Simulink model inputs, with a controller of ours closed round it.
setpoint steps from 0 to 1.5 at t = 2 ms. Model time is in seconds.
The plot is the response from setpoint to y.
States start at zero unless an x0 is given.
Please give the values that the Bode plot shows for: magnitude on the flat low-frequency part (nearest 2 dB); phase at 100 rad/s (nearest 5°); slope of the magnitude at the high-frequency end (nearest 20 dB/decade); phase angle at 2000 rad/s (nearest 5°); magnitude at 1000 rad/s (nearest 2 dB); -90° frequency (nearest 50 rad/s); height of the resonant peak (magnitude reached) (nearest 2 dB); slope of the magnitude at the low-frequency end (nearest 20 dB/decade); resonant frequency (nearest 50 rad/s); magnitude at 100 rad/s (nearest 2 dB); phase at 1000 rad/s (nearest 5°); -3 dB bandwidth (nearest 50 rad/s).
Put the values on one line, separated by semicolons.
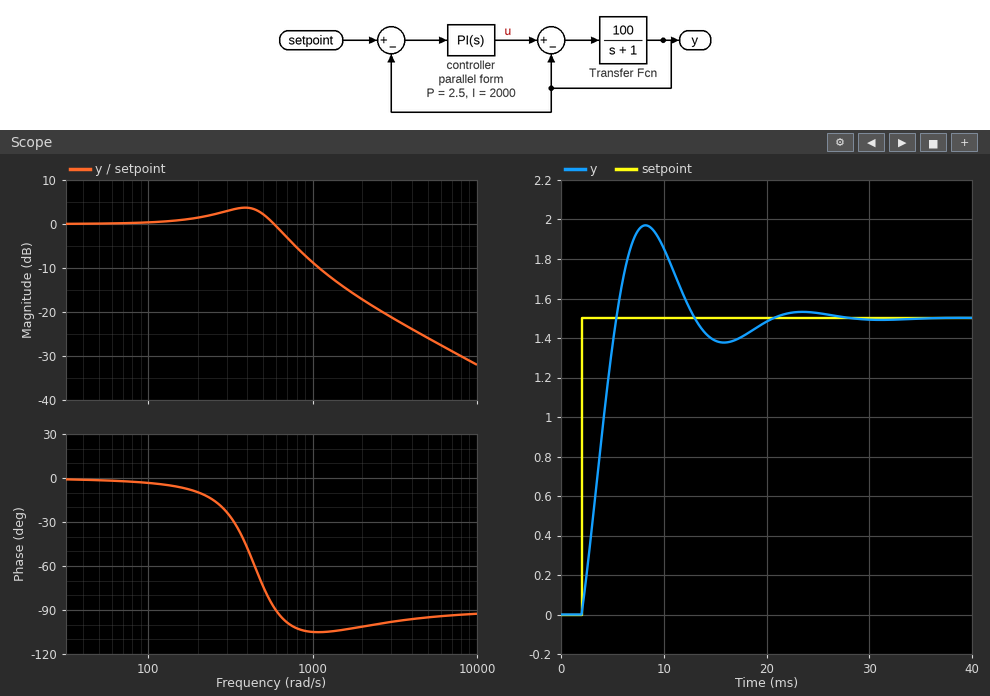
0 dB; -5°; -20 dB/decade; -100°; -8 dB; 600 rad/s; 4 dB; 0 dB/decade; 400 rad/s; 0 dB; -105°; 700 rad/s
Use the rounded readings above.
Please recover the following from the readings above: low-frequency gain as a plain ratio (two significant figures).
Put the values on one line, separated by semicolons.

1.0
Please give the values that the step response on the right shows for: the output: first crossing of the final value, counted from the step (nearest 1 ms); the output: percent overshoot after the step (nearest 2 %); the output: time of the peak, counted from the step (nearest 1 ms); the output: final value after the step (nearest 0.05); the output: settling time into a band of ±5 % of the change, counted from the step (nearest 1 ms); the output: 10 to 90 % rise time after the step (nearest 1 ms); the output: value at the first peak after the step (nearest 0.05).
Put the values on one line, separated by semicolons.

3 ms; 32 %; 6 ms; 1.50; 16 ms; 3 ms; 1.95
